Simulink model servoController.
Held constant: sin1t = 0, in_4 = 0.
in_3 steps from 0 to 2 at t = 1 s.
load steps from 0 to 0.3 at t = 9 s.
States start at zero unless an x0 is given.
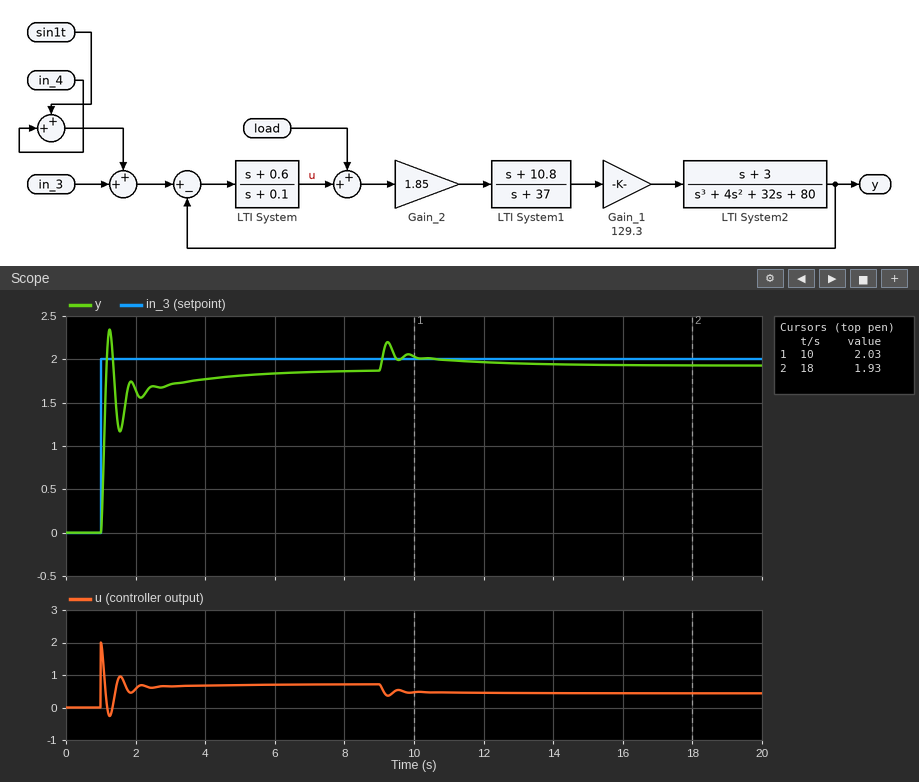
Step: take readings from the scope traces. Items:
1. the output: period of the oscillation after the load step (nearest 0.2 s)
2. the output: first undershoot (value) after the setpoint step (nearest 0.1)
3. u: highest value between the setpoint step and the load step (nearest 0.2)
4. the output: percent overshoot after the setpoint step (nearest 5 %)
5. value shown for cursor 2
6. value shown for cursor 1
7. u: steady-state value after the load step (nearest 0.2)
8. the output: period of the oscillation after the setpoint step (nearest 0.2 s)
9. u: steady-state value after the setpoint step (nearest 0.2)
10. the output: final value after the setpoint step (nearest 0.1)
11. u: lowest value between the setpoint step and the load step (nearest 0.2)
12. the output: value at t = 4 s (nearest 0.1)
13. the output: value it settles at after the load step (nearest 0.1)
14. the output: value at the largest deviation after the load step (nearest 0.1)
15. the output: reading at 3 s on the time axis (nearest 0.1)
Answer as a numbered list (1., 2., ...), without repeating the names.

1. 0.6 s
2. 1.2
3. 2.0
4. 25 %
5. 1.93
6. 2.03
7. 0.4
8. 0.6 s
9. 0.8
10. 1.9
11. -0.2
12. 1.8
13. 1.9
14. 2.2
15. 1.7
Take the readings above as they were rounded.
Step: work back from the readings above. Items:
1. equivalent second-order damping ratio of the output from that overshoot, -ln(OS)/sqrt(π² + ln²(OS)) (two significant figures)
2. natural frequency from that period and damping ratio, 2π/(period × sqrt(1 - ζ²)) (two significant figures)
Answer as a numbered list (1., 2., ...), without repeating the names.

1. 0.40
2. 11 rad/s
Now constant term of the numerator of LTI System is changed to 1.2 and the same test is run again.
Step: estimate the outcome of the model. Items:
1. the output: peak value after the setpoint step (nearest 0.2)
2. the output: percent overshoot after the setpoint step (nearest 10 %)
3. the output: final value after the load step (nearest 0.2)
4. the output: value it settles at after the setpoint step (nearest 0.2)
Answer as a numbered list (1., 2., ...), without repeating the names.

1. 2.4
2. 30 %
3. 2.0
4. 2.0
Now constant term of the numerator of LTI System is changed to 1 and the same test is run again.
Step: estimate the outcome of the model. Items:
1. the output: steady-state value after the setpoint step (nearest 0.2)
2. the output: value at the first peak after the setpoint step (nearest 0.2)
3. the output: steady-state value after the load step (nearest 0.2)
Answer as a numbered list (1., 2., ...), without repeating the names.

1. 2.0
2. 2.4
3. 2.0
